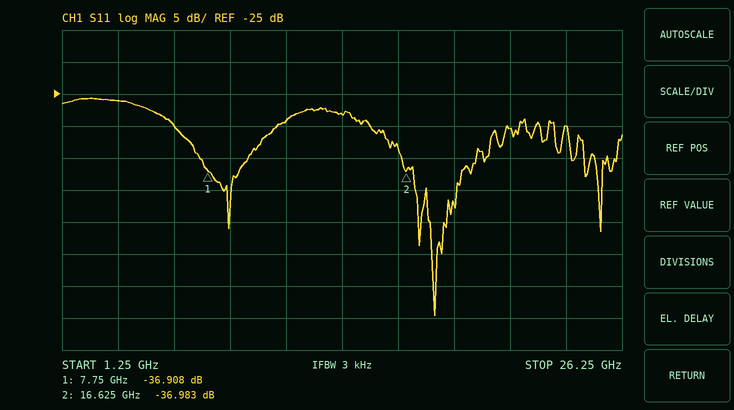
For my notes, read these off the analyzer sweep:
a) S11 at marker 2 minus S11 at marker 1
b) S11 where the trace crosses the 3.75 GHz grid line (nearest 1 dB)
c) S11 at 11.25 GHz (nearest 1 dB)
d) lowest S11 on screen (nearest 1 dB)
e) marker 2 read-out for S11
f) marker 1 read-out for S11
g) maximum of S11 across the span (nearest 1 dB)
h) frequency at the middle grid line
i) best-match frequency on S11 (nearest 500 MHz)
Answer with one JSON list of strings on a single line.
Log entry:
["-0.075 dB", "-26 dB", "-29 dB", "-60 dB", "-36.983 dB", "-36.908 dB", "-26 dB", "13.75 GHz", "18.0 GHz"]
